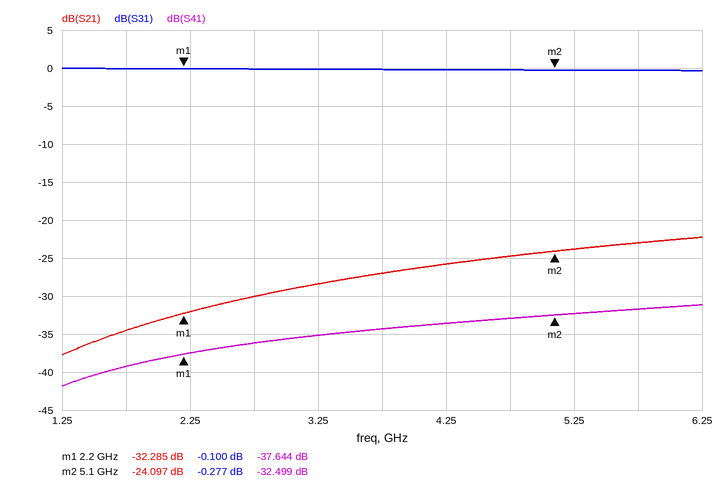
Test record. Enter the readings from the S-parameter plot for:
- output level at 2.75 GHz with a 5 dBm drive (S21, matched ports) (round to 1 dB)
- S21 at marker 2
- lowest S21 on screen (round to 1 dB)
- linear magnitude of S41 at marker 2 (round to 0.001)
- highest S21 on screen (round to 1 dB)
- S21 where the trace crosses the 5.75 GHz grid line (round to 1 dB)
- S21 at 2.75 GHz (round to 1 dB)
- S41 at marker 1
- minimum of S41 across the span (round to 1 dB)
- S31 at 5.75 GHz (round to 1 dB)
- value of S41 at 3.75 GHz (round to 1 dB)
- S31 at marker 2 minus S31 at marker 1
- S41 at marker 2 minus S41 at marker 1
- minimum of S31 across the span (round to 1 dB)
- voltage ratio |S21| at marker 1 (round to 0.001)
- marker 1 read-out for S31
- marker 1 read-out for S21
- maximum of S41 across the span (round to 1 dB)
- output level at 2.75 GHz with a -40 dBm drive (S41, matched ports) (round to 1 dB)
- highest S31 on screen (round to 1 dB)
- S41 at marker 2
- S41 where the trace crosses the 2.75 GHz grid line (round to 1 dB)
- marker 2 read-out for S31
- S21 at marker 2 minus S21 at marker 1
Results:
-25 dBm
-24.097 dB
-38 dB
0.024
-22 dB
-23 dB
-30 dB
-37.644 dB
-42 dB
0 dB
-34 dB
-0.177 dB
5.145 dB
0 dB
0.024
-0.100 dB
-32.285 dB
-31 dB
-76 dBm
0 dB
-32.499 dB
-36 dB
-0.277 dB
8.188 dB
